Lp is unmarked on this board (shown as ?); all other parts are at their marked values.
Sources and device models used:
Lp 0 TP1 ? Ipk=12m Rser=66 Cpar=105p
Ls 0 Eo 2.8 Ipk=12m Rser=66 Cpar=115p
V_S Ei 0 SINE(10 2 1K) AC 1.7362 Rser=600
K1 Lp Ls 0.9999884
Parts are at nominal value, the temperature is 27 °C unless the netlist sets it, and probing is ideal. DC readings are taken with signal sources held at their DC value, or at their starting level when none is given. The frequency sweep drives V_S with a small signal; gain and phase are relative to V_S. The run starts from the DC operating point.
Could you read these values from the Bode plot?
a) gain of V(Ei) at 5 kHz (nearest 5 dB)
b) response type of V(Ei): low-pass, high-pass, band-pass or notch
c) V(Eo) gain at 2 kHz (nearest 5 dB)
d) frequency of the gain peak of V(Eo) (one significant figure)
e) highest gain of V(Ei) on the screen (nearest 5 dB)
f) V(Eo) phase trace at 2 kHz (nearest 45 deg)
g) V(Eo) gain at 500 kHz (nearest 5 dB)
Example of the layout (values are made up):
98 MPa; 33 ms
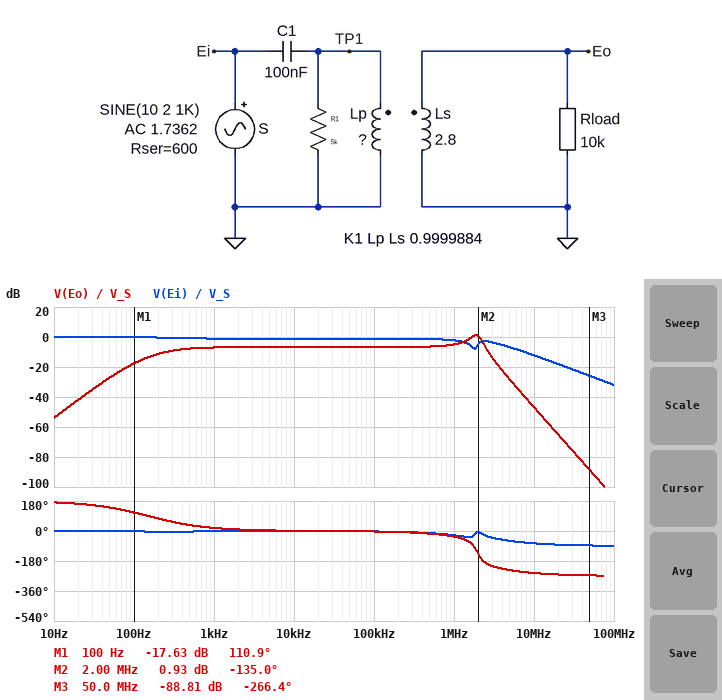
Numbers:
0 dB; low-pass; -5 dB; 2 MHz; 0 dB; 0 deg; -5 dB
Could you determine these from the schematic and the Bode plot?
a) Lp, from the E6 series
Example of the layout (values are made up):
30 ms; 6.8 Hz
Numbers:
10 H
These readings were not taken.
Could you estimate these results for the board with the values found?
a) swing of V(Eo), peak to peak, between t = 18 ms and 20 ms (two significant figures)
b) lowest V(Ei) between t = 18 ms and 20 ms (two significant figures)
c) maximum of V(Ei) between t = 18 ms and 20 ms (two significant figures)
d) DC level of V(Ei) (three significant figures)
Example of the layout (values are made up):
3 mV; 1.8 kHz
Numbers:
1.8 V; 8.2 V; 12 V; 10.0 V
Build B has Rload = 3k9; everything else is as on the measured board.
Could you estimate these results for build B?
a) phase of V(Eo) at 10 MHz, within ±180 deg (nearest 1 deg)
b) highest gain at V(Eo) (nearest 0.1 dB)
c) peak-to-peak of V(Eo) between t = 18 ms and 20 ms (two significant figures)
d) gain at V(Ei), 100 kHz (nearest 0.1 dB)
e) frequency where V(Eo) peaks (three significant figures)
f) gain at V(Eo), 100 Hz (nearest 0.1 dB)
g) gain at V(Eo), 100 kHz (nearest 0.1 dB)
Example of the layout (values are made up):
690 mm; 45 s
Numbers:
109 deg; -1.1 dB; 1.7 V; -1.3 dB; 1.87 MHz; -19.0 dB; -7.0 dB
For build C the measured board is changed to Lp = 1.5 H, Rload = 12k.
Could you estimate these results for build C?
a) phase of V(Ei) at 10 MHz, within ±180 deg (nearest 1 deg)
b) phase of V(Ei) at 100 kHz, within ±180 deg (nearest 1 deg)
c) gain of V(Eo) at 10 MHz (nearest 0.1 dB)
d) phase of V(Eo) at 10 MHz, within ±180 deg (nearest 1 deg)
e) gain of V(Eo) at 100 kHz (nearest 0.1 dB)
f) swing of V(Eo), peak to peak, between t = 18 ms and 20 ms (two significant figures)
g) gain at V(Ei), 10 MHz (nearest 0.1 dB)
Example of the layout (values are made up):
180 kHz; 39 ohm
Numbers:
-73 deg; -6 deg; -38.1 dB; 111 deg; 0.9 dB; 4.4 V; -11.7 dB
